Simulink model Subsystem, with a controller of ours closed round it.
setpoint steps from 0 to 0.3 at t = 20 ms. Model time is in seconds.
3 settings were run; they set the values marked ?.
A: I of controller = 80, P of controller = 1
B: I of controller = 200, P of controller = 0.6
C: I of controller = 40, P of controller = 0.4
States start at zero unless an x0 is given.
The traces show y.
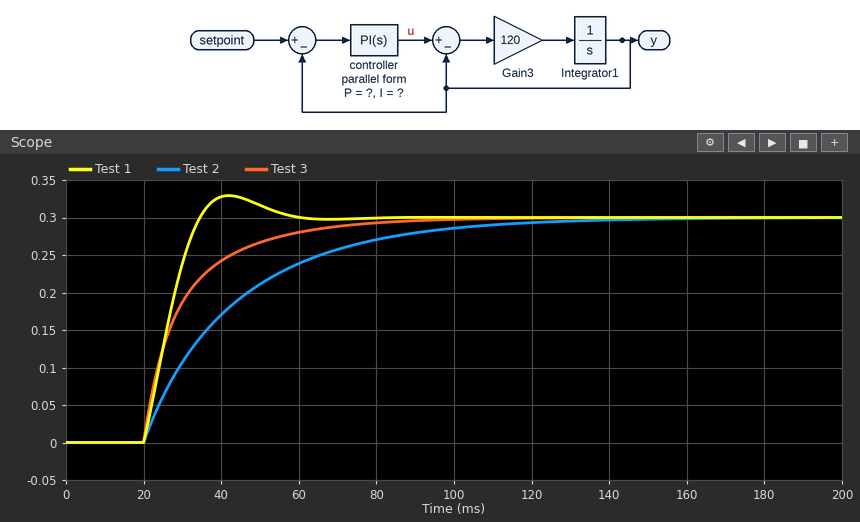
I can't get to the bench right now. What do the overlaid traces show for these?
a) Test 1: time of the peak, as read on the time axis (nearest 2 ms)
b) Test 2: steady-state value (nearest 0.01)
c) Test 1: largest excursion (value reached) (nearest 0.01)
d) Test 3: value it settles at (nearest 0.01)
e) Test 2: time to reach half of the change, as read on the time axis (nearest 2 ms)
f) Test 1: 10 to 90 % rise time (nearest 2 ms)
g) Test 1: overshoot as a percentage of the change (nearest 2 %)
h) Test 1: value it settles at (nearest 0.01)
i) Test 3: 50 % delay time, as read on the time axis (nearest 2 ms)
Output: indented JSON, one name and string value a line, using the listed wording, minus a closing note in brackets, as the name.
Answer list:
{
  "Test 1: time of the peak, as read on the time axis": "42 ms",
  "Test 2: steady-state value": "0.30",
  "Test 1: largest excursion (value reached)": "0.33",
  "Test 3: value it settles at": "0.30",
  "Test 2: time to reach half of the change, as read on the time axis": "36 ms",
  "Test 1: 10 to 90 % rise time": "10 ms",
  "Test 1: overshoot as a percentage of the change": "10 %",
  "Test 1: value it settles at": "0.30",
  "Test 3: 50 % delay time, as read on the time axis": "26 ms"
}
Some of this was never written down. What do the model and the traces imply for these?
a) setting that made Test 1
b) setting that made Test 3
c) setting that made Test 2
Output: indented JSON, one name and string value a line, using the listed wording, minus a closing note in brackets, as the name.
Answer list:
{
  "setting that made Test 1": "B",
  "setting that made Test 3": "A",
  "setting that made Test 2": "C"
}
